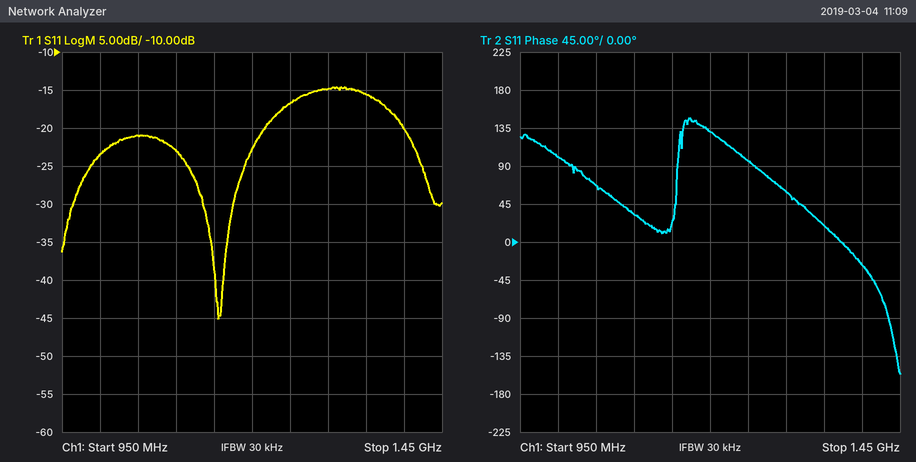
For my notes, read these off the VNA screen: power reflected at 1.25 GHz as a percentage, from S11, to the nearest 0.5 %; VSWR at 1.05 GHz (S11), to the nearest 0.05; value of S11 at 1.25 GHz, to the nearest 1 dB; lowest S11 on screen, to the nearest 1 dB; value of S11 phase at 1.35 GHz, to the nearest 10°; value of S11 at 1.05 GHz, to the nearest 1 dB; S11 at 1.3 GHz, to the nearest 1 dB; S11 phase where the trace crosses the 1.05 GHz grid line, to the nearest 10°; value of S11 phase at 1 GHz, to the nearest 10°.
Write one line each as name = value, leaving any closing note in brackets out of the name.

power reflected at 1.25 GHz as a percentage, from S11, to the nearest 0.5 % = 2.0 %
VSWR at 1.05 GHz (S11), to the nearest 0.05 = 1.20
value of S11 at 1.25 GHz, to the nearest 1 dB = -17 dB
lowest S11 on screen, to the nearest 1 dB = -45 dB
value of S11 phase at 1.35 GHz, to the nearest 10° = 20°
value of S11 at 1.05 GHz, to the nearest 1 dB = -21 dB
S11 at 1.3 GHz, to the nearest 1 dB = -15 dB
S11 phase where the trace crosses the 1.05 GHz grid line, to the nearest 10° = 70°
value of S11 phase at 1 GHz, to the nearest 10° = 100°
